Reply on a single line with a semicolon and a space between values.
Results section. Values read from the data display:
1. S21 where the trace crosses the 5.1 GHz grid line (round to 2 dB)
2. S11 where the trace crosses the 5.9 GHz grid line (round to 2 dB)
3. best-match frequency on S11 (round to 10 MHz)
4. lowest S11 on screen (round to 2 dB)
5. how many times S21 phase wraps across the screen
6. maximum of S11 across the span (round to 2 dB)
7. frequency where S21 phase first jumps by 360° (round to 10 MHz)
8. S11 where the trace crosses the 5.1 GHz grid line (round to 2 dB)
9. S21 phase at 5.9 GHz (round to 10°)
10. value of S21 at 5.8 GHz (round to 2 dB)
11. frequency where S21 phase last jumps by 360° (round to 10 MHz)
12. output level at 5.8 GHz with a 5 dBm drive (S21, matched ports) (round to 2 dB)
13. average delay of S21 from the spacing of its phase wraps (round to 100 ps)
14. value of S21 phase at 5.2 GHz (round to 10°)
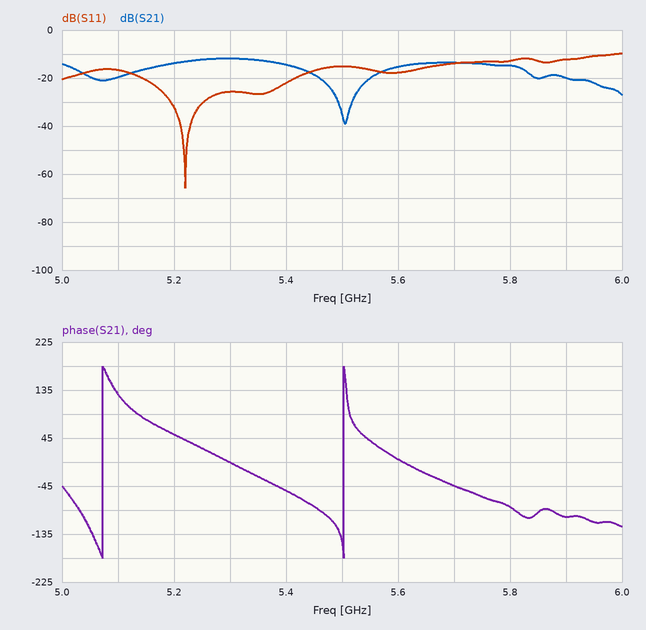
-20 dB; -12 dB; 5.22 GHz; -66 dB; 2; -10 dB; 5.07 GHz; -16 dB; -100°; -14 dB; 5.50 GHz; -10 dBm; 2.3 ns; 50°
